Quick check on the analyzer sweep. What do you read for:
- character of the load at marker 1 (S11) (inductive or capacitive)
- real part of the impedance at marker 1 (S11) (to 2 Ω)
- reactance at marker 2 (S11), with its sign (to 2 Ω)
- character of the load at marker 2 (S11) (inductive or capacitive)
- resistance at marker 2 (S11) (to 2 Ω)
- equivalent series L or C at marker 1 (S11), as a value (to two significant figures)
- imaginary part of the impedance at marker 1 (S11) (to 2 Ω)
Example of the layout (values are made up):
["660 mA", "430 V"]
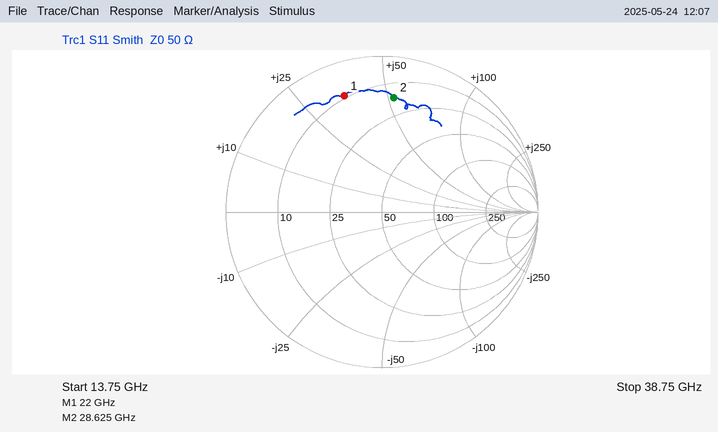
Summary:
["inductive", "10 Ω", "+52 Ω", "inductive", "16 Ω", "260 pH", "+36 Ω"]
